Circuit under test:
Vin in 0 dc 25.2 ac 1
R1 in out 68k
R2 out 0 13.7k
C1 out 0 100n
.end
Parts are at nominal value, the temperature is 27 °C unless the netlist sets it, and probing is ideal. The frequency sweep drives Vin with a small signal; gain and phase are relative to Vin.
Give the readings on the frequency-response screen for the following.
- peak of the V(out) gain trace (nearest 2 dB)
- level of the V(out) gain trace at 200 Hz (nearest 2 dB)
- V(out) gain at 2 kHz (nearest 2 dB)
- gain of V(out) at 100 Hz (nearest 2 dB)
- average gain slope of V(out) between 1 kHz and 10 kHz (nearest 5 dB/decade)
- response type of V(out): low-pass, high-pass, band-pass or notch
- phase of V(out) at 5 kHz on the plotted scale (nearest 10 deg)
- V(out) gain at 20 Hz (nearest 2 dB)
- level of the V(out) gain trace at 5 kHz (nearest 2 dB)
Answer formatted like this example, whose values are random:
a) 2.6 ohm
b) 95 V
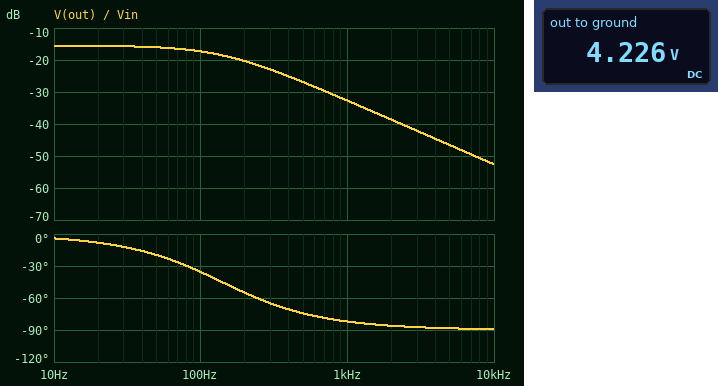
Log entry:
a) -16 dB
b) -20 dB
c) -38 dB
d) -18 dB
e) -20 dB/decade
f) low-pass
g) -90 deg
h) -16 dB
i) -46 dB
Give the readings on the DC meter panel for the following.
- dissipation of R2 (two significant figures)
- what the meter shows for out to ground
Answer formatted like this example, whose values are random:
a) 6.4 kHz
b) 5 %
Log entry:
a) 1.3 mW
b) 4.226 V
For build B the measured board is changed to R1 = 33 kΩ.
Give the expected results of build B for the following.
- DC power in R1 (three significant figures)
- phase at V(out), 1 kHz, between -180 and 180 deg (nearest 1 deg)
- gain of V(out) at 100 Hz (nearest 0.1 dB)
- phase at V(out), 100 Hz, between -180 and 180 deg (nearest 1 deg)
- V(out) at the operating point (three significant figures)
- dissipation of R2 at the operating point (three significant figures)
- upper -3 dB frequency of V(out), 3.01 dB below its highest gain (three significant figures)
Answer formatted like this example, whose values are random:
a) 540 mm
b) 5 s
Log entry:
a) 9.61 mW
b) -81 deg
c) -12.0 dB
d) -31 deg
e) 7.39 V
f) 3.99 mW
g) 164 Hz
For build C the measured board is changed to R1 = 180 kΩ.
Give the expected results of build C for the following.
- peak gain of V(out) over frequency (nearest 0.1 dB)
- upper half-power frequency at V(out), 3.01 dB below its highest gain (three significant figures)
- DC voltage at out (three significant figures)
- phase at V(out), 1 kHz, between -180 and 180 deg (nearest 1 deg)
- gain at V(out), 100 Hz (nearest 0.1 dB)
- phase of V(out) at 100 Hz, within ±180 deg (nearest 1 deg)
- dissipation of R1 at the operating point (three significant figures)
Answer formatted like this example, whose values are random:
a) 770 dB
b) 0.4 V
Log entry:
a) -23.0 dB
b) 125 Hz
c) 1.78 V
d) -83 deg
e) -25.2 dB
f) -39 deg
g) 3.05 mW
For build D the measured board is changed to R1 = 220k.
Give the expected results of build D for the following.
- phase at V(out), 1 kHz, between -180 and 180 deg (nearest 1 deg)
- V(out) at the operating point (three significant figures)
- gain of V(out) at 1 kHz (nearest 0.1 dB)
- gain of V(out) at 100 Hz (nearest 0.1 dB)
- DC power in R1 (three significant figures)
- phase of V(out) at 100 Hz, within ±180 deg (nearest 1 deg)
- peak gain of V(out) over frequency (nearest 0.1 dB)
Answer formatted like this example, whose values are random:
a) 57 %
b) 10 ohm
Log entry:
a) -83 deg
b) 1.48 V
c) -42.9 dB
d) -26.8 dB
e) 2.56 mW
f) -39 deg
g) -24.6 dB
